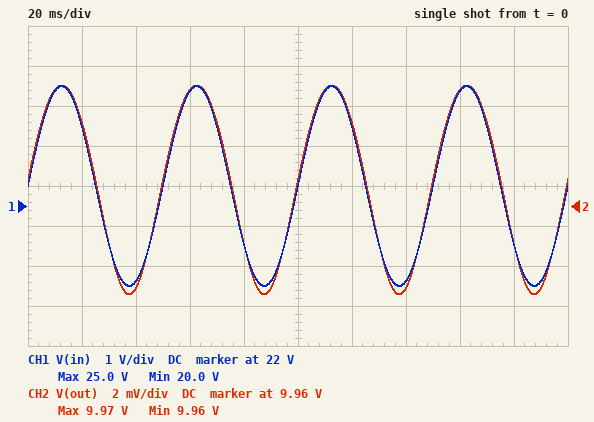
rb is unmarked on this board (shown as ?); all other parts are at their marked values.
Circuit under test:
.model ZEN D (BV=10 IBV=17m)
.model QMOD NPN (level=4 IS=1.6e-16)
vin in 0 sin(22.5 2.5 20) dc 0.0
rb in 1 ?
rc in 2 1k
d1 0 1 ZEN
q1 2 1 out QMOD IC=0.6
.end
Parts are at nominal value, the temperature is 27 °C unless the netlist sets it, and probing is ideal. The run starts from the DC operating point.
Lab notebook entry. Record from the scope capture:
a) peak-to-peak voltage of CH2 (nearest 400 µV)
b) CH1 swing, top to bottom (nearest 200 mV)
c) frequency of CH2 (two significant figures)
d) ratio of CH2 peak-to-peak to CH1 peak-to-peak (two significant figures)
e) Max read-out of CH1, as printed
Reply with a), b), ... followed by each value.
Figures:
a) 10.4 mV
b) 5.0 V
c) 20 Hz
d) 0.0021
e) 25.0 V
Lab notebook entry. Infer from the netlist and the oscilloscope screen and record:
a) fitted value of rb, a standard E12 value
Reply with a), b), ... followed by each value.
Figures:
a) 3.3 kΩ
